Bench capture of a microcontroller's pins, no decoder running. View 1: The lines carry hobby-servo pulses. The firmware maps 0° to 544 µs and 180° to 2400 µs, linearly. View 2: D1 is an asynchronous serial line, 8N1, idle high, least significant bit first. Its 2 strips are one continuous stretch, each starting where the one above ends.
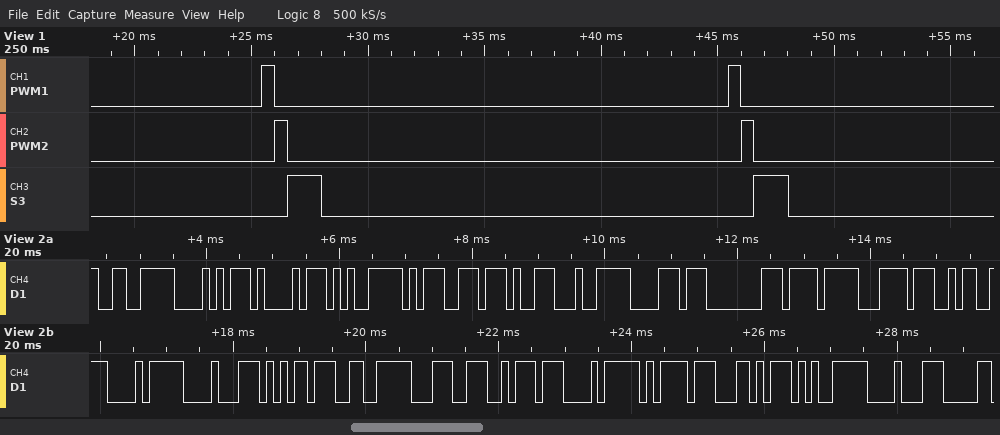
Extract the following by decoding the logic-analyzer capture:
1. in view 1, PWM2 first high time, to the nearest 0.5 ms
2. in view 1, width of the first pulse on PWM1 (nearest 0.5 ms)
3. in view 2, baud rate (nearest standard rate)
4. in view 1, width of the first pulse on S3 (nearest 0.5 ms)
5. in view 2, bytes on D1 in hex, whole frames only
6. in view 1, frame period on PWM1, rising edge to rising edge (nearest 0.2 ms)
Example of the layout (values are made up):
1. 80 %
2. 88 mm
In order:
1. 0.5 ms
2. 0.5 ms
3. 9600 baud
4. 1.5 ms
5. E6 A8 A1 E5 9D 97 E4 B8 80 EF BC 9A E8 88 B5 E6 9C BA E8 BD AC E5 88
6. 20.0 ms
